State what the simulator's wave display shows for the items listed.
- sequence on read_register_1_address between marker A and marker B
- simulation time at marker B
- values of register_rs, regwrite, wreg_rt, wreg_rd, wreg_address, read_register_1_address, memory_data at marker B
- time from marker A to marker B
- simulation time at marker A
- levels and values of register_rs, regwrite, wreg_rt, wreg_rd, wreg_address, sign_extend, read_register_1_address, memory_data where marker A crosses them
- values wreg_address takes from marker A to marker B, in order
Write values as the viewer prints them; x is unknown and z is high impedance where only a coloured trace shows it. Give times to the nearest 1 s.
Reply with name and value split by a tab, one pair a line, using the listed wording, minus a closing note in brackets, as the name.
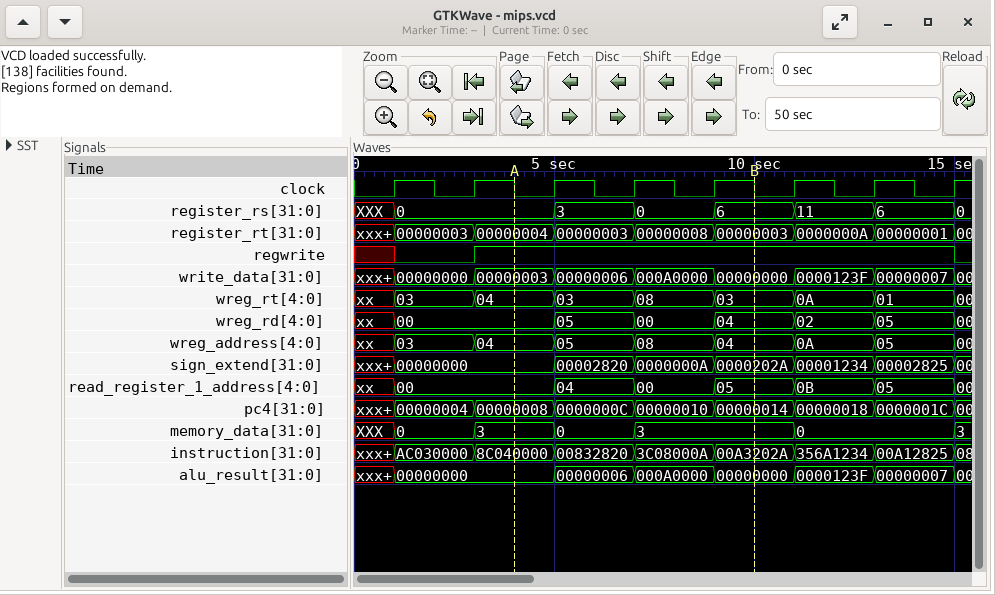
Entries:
sequence on read_register_1_address between marker A and marker B	00, 04, 00, 05
simulation time at marker B	10 s
values of register_rs, regwrite, wreg_rt, wreg_rd, wreg_address, read_register_1_address, memory_data at marker B	register_rs=6, regwrite=1, wreg_rt=03, wreg_rd=04, wreg_address=04, read_register_1_address=05, memory_data=3
time from marker A to marker B	6 s
simulation time at marker A	4 s
levels and values of register_rs, regwrite, wreg_rt, wreg_rd, wreg_address, sign_extend, read_register_1_address, memory_data where marker A crosses them	register_rs=0, regwrite=1, wreg_rt=04, wreg_rd=00, wreg_address=04, sign_extend=00000000, read_register_1_address=00, memory_data=3
values wreg_address takes from marker A to marker B, in order	04, 05, 08, 04
